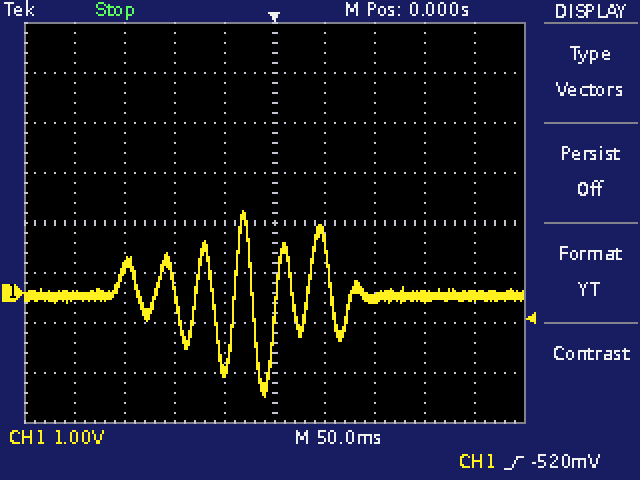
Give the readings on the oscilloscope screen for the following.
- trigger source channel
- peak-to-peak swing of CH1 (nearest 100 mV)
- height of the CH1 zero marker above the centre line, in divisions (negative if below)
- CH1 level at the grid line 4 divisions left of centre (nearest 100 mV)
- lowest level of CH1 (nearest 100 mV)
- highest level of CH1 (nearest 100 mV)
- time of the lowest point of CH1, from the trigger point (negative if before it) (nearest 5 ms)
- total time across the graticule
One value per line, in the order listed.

CH1
3.7 V
-1.4 div
-100 mV
-2.1 V
1.6 V
-10 ms
500 ms
